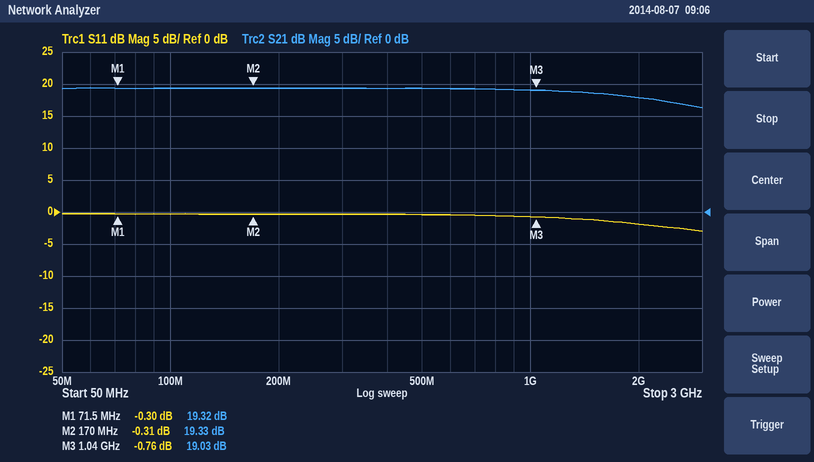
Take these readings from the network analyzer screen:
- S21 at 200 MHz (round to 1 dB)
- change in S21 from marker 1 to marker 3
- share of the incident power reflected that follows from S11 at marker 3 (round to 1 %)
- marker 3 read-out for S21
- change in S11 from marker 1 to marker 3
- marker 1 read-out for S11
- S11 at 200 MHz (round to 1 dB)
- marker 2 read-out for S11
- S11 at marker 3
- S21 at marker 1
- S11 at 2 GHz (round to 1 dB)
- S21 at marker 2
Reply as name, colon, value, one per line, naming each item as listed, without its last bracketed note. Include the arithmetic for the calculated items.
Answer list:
S21 at 200 MHz: 19 dB
change in S21 from marker 1 to marker 3: 19.03 − (19.32) = -0.29 dB
share of the incident power reflected that follows from S11 at marker 3: 10^(-0.76/10) ≈ 84 %
marker 3 read-out for S21: 19.03 dB
change in S11 from marker 1 to marker 3: -0.76 − (-0.3) = -0.46 dB
marker 1 read-out for S11: -0.30 dB
S11 at 200 MHz: 0 dB
marker 2 read-out for S11: -0.31 dB
S11 at marker 3: -0.76 dB
S21 at marker 1: 19.32 dB
S11 at 2 GHz: -2 dB
S21 at marker 2: 19.33 dB
